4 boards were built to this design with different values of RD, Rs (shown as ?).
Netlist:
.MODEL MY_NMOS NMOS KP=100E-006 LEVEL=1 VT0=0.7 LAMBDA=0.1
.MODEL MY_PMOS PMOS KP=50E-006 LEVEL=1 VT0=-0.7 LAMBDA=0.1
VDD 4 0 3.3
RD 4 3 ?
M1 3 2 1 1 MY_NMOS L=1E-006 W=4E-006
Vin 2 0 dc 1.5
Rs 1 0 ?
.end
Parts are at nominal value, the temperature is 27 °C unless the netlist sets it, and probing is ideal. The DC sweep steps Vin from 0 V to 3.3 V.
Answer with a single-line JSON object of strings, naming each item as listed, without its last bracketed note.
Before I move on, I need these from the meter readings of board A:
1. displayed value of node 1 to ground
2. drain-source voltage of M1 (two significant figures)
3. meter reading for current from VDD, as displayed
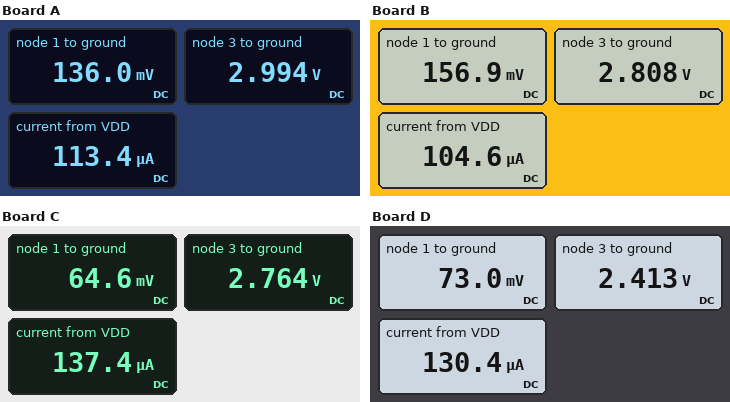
{"displayed value of node 1 to ground": "136.0 mV", "drain-source voltage of M1": "2.9 V", "meter reading for current from VDD, as displayed": "113.4 µA"}
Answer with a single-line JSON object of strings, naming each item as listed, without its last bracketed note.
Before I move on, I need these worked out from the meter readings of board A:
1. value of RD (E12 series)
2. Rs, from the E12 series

{"value of RD": "2.7 kΩ", "Rs, from the E12 series": "1.2 kΩ"}
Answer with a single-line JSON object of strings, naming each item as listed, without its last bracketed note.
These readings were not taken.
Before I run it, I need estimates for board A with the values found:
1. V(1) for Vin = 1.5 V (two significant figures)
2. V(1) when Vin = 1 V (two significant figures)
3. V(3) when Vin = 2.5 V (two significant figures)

{"V(1) for Vin = 1.5 V": "140 mV", "V(1) when Vin = 1 V": "24 mV", "V(3) when Vin = 2.5 V": "2.2 V"}
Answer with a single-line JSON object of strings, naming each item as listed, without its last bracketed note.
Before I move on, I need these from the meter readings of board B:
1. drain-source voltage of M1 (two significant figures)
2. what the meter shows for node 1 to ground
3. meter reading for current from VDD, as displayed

{"drain-source voltage of M1": "2.7 V", "what the meter shows for node 1 to ground": "156.9 mV", "meter reading for current from VDD, as displayed": "104.6 µA"}
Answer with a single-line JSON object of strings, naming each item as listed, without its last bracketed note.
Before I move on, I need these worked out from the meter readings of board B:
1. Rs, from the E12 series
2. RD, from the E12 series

{"Rs, from the E12 series": "1.5 kΩ", "RD, from the E12 series": "4.7 kΩ"}
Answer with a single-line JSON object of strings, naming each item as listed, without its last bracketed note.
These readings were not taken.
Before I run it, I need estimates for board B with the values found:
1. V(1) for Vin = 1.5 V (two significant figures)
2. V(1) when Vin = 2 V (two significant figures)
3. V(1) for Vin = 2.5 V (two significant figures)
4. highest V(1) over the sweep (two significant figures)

{"V(1) for Vin = 1.5 V": "160 mV", "V(1) when Vin = 2 V": "330 mV", "V(1) for Vin = 2.5 V": "530 mV", "highest V(1) over the sweep": "650 mV"}
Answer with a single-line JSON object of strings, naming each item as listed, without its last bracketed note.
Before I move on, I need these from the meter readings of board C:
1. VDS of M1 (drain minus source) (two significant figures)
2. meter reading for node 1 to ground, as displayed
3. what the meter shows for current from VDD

{"VDS of M1 (drain minus source)": "2.7 V", "meter reading for node 1 to ground, as displayed": "64.6 mV", "what the meter shows for current from VDD": "137.4 µA"}
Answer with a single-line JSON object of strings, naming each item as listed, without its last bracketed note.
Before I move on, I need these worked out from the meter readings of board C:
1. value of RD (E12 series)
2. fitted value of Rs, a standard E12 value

{"value of RD": "3.9 kΩ", "fitted value of Rs, a standard E12 value": "470 Ω"}
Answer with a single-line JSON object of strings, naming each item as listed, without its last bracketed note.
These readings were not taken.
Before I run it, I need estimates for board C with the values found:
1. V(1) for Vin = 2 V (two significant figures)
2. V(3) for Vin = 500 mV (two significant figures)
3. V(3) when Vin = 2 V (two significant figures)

{"V(1) for Vin = 2 V": "150 mV", "V(3) for Vin = 500 mV": "3.3 V", "V(3) when Vin = 2 V": "2.1 V"}
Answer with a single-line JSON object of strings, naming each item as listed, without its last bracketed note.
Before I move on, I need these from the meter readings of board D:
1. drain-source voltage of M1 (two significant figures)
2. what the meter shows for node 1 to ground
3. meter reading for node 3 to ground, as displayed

{"drain-source voltage of M1": "2.3 V", "what the meter shows for node 1 to ground": "73.0 mV", "meter reading for node 3 to ground, as displayed": "2.413 V"}
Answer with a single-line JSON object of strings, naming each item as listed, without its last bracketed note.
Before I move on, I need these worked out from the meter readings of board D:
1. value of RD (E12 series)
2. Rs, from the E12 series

{"value of RD": "6.8 kΩ", "Rs, from the E12 series": "560 Ω"}
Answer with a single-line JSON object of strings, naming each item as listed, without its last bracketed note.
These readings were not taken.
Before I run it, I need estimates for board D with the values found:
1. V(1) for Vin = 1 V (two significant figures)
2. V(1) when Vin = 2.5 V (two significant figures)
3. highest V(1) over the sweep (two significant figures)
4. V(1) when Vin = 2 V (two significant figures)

{"V(1) for Vin = 1 V": "12 mV", "V(1) when Vin = 2.5 V": "200 mV", "highest V(1) over the sweep": "220 mV", "V(1) when Vin = 2 V": "160 mV"}
